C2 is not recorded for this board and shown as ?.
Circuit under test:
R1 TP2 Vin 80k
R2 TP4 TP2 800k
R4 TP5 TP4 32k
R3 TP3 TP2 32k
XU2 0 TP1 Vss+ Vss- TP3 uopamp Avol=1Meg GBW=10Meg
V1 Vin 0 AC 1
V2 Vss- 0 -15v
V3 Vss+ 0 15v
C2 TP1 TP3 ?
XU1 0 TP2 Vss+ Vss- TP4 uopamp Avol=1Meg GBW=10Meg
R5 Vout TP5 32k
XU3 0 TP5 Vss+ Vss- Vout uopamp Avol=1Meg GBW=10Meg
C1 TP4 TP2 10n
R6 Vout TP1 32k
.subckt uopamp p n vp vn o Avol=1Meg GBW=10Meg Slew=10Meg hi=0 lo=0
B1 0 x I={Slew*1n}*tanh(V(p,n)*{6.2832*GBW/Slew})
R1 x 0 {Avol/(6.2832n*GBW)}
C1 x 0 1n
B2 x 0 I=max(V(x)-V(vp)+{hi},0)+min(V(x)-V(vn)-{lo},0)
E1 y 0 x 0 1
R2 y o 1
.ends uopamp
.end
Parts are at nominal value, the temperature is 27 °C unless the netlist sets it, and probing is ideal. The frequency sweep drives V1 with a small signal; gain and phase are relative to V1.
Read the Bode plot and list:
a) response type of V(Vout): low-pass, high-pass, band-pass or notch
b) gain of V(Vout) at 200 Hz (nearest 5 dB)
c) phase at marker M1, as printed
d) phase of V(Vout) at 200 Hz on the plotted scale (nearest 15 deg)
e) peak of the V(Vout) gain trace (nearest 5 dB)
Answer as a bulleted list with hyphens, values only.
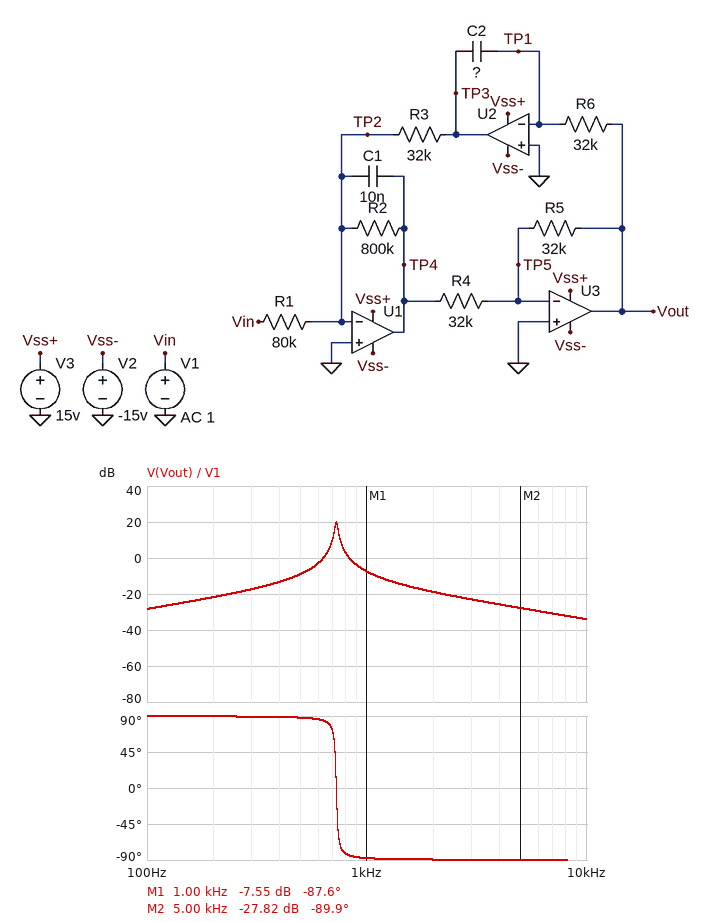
- band-pass
- -20 dB
- -87.6 deg
- 90 deg
- 20 dB
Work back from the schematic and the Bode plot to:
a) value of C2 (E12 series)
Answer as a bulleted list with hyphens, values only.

- 4.7 nF
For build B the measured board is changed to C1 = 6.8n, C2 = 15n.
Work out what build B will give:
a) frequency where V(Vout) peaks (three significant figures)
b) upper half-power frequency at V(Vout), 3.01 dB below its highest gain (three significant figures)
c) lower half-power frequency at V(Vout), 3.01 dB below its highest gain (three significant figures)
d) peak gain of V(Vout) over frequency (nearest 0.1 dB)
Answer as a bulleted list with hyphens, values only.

- 492 Hz
- 507 Hz
- 478 Hz
- 20.0 dB
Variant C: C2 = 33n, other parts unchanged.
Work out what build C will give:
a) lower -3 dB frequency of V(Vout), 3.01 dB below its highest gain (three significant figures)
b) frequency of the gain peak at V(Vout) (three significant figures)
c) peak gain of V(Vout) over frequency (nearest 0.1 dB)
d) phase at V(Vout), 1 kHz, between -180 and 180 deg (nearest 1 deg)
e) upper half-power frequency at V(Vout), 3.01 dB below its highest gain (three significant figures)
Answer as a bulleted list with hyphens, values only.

- 264 Hz
- 274 Hz
- 20.0 dB
- -89 deg
- 284 Hz
